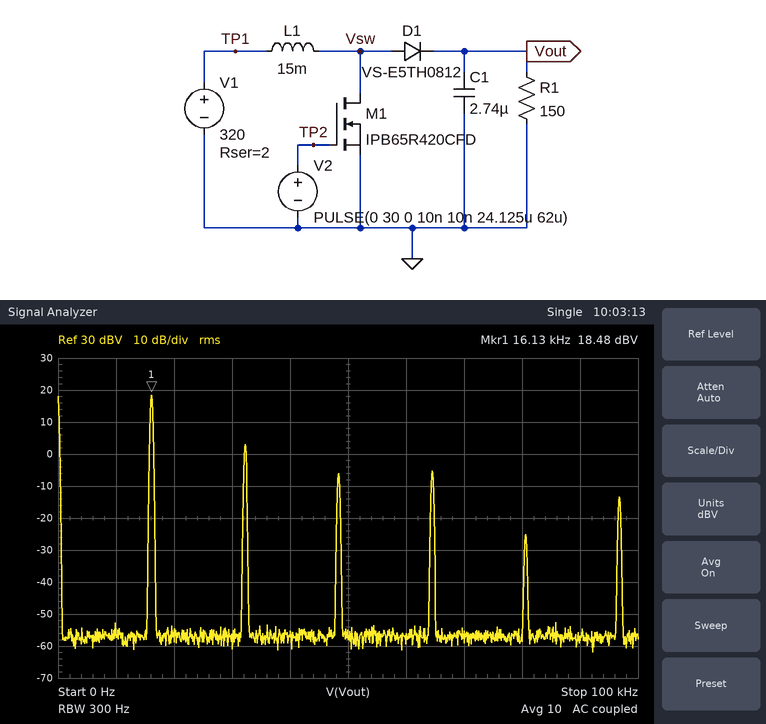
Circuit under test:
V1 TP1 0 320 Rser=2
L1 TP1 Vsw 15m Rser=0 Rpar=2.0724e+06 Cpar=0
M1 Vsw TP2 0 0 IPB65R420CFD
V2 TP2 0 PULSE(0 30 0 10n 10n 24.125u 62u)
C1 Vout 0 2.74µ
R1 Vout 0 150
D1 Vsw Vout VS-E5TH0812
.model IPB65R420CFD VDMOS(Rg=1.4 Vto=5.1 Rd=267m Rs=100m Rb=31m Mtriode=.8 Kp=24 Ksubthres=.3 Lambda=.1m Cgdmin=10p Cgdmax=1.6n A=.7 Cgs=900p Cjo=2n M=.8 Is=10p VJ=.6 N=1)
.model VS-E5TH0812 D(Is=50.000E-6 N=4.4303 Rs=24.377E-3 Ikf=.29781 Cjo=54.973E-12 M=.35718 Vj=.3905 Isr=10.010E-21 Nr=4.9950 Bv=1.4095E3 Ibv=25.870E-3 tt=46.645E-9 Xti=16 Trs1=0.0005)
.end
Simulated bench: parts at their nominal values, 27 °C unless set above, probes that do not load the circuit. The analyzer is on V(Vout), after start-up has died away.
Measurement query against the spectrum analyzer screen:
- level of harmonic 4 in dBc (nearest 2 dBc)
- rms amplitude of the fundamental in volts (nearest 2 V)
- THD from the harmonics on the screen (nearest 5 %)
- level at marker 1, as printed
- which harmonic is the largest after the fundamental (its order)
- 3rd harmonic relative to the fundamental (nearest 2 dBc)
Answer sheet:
-24 dBc
8 V
20 %
18.48 dBV
2
-24 dBc
